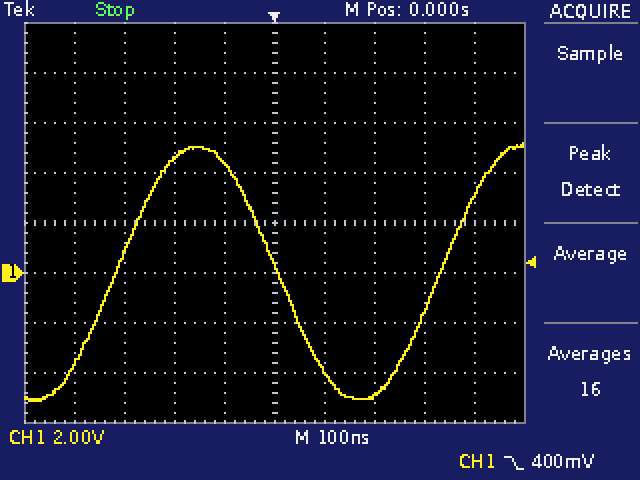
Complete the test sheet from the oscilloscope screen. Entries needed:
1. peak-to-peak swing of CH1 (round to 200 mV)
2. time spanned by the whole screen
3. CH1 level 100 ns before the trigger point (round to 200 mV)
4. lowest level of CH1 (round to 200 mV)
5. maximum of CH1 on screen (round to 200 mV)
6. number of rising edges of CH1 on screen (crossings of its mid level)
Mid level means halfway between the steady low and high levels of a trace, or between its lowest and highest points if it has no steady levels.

10.4 V
1 µs
4.4 V
-5.2 V
5.2 V
2
